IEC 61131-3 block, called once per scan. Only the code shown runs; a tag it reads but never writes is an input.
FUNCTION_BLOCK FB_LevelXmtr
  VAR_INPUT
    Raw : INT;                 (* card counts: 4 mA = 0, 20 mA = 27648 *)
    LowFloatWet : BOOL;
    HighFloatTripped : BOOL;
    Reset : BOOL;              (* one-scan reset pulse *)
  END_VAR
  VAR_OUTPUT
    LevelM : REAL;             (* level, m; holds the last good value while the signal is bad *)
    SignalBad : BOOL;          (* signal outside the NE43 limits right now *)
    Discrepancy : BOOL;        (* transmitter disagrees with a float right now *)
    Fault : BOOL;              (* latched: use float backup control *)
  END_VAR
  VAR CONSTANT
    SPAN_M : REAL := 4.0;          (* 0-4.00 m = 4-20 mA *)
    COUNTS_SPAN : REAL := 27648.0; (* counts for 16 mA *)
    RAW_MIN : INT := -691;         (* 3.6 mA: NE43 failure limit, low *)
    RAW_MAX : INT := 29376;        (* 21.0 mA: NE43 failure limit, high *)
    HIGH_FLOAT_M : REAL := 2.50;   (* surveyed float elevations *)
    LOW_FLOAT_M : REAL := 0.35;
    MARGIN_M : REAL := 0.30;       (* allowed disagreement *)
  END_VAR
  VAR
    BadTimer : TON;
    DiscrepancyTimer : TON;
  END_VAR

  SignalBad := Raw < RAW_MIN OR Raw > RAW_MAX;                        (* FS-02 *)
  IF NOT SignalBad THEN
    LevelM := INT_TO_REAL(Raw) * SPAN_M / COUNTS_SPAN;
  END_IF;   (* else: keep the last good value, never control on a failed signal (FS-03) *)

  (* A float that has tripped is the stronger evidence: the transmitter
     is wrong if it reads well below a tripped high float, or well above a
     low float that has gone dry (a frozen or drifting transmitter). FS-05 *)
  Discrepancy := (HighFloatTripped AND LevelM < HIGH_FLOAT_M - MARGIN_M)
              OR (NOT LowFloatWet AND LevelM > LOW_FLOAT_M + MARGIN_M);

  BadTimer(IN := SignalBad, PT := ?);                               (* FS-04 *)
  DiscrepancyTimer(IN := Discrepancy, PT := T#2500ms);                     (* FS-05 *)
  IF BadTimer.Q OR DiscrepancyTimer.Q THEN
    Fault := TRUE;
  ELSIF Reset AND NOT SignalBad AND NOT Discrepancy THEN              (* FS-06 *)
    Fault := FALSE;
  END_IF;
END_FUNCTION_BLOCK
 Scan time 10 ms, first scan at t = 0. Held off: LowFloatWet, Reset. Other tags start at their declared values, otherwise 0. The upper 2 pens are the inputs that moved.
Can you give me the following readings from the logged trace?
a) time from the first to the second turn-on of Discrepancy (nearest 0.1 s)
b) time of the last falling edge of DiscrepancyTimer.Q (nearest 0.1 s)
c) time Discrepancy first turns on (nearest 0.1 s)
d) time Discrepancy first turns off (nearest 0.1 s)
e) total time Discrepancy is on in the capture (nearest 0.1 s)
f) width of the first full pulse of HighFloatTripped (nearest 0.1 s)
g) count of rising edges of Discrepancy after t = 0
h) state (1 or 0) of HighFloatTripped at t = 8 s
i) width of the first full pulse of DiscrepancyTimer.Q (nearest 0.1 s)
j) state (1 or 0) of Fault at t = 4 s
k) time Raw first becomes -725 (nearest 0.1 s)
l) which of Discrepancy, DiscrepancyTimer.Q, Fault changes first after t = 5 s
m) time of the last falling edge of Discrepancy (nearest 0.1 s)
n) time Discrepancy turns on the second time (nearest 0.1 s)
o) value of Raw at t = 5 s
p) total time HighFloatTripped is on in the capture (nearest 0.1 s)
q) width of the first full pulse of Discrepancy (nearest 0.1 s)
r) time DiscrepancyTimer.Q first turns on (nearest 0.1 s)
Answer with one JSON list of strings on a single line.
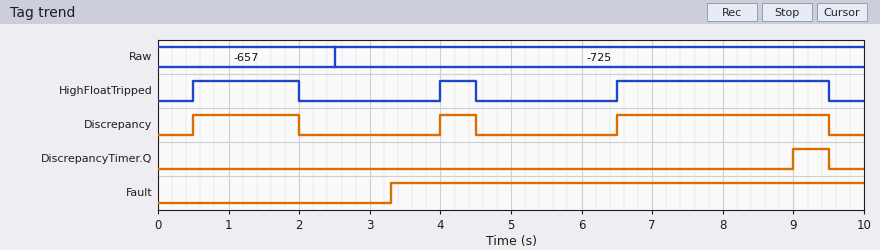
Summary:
["3.5 s", "9.5 s", "0.5 s", "2.0 s", "5.0 s", "1.5 s", "3", "1", "0.5 s", "1", "2.5 s", "Discrepancy", "9.5 s", "4.0 s", "-725", "5.0 s", "1.5 s", "9.0 s"]
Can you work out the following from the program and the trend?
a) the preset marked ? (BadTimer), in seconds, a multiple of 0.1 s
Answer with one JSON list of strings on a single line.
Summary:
["0.8 s"]
